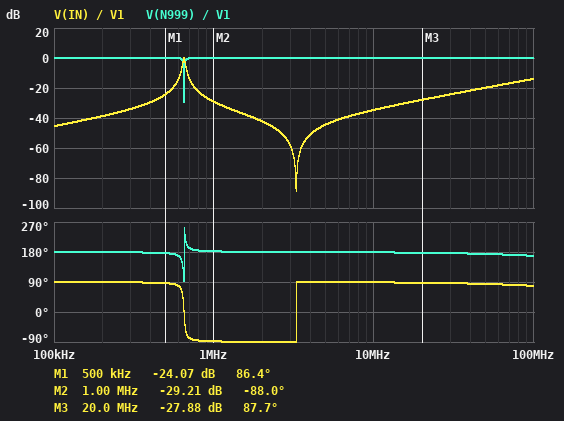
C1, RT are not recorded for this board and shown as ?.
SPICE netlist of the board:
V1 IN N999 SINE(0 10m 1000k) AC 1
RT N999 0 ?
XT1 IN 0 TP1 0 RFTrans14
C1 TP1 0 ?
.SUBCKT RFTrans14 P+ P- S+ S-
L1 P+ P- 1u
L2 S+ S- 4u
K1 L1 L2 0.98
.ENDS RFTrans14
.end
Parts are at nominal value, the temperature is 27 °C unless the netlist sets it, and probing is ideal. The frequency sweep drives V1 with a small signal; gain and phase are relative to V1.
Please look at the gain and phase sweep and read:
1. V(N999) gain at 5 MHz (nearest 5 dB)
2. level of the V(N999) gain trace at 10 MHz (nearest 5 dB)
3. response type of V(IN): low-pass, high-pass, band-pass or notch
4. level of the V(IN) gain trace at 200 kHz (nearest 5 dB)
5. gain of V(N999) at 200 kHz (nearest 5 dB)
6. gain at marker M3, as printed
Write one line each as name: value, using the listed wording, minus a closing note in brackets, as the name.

V(N999) gain at 5 MHz: 0 dB
level of the V(N999) gain trace at 10 MHz: 0 dB
response type of V(IN): low-pass, high-pass, band-pass or notch: band-pass
level of the V(IN) gain trace at 200 kHz: -40 dB
gain of V(N999) at 200 kHz: 0 dB
gain at marker M3, as printed: -27.88 dB
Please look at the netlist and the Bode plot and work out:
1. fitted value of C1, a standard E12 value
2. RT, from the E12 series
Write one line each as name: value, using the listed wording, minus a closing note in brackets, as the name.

fitted value of C1, a standard E12 value: 15 nF
RT, from the E12 series: 120 Ω
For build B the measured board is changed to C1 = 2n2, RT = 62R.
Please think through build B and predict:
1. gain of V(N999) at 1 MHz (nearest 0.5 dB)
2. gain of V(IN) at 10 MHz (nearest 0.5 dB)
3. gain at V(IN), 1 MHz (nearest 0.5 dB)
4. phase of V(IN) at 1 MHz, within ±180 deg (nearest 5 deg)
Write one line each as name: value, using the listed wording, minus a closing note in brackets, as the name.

gain of V(N999) at 1 MHz: 0 dB
gain of V(IN) at 10 MHz: -39.0 dB
gain at V(IN), 1 MHz: -16.5 dB
phase of V(IN) at 1 MHz, within ±180 deg: 80 deg
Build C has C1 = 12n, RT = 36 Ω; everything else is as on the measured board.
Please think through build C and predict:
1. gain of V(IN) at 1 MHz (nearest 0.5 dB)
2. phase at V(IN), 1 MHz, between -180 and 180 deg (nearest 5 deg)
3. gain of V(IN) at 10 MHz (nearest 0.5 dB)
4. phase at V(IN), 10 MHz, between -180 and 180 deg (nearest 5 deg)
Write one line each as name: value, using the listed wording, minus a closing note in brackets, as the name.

gain of V(IN) at 1 MHz: -15.0 dB
phase at V(IN), 1 MHz, between -180 and 180 deg: -80 deg
gain of V(IN) at 10 MHz: -24.5 dB
phase at V(IN), 10 MHz, between -180 and 180 deg: 85 deg
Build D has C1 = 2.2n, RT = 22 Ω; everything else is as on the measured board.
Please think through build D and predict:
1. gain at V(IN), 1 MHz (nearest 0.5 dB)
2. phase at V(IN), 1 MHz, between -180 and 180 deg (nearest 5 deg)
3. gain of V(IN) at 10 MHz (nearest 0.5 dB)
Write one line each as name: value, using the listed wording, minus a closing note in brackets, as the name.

gain at V(IN), 1 MHz: -8.0 dB
phase at V(IN), 1 MHz, between -180 and 180 deg: 65 deg
gain of V(IN) at 10 MHz: -30.0 dB
